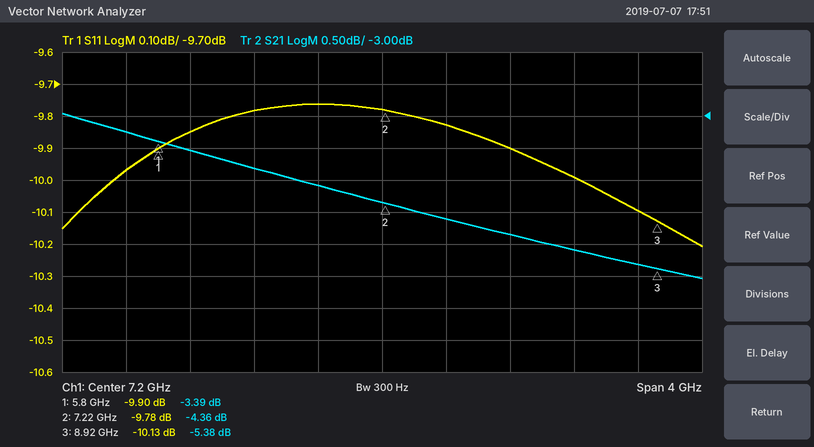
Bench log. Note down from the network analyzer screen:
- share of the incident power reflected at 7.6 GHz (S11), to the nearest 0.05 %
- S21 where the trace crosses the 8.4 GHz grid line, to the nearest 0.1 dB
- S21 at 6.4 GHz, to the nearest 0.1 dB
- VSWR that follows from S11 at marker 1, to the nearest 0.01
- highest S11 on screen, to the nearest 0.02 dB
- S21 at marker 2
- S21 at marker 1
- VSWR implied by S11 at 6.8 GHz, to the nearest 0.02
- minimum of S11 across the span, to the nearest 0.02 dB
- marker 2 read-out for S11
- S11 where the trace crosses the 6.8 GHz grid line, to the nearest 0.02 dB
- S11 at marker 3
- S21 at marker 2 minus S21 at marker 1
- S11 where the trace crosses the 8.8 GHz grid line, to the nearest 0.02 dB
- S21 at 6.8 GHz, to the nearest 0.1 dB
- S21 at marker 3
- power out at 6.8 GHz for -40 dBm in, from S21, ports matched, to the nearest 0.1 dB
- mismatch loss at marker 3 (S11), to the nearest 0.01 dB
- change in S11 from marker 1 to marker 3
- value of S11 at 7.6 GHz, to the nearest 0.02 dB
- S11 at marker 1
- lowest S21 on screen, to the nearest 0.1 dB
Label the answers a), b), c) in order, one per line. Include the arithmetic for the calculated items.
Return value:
a) 10^(-9.82/10) ≈ 10.40 %
b) -5.1 dB
c) -3.8 dB
d) (1 + 0.3199)/(1 − 0.3199) ≈ 1.94
e) -9.76 dB
f) -4.36 dB
g) -3.39 dB
h) |Γ| = 10^(-9.76/20) = 0.3251; VSWR = (1 + 0.3251)/(1 − 0.3251) ≈ 1.96
i) -10.20 dB
j) -9.78 dB
k) -9.76 dB
l) -10.13 dB
m) -4.36 − (-3.39) = -0.97 dB
n) -10.10 dB
o) -4.1 dB
p) -5.38 dB
q) -40 dBm + (-4.1 dB) = -44.1 dBm
r) −10 log10(1 − 10^(-10.13/10)) ≈ 0.44 dB
s) -10.13 − (-9.9) = -0.23 dB
t) -9.82 dB
u) -9.90 dB
v) -5.5 dB
